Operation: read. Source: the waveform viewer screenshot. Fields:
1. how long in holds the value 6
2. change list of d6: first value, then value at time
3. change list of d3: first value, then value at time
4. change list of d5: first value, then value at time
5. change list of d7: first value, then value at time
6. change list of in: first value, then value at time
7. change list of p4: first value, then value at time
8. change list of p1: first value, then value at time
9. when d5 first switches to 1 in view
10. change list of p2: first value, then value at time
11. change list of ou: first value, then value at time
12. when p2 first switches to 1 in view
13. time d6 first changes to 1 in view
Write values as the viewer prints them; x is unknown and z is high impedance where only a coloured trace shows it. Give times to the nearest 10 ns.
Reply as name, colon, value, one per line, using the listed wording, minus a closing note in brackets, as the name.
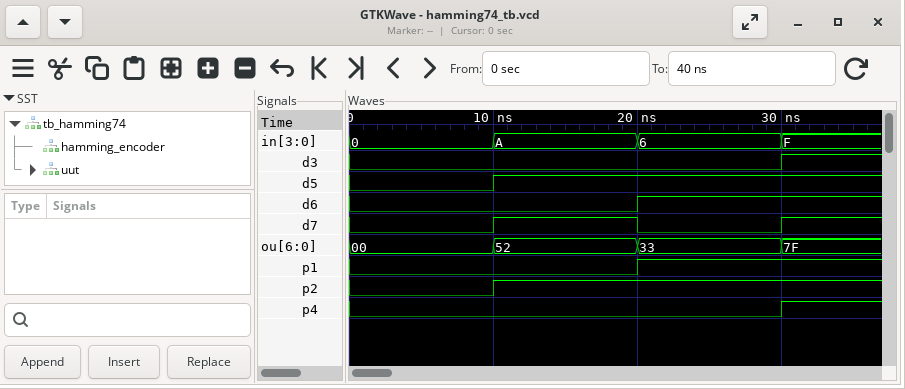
how long in holds the value 6: 10 ns
change list of d6: first value, then value at time: 0, 1 at 20 ns
change list of d3: first value, then value at time: 0, 1 at 30 ns
change list of d5: first value, then value at time: 0, 1 at 10 ns
change list of d7: first value, then value at time: 0, 1 at 10 ns, 0 at 20 ns, 1 at 30 ns
change list of in: first value, then value at time: 0, A at 10 ns, 6 at 20 ns, F at 30 ns
change list of p4: first value, then value at time: 0, 1 at 30 ns
change list of p1: first value, then value at time: 0, 1 at 20 ns
when d5 first switches to 1 in view: 10 ns
change list of p2: first value, then value at time: 0, 1 at 10 ns
change list of ou: first value, then value at time: 00, 52 at 10 ns, 33 at 20 ns, 7F at 30 ns
when p2 first switches to 1 in view: 10 ns
time d6 first changes to 1 in view: 20 ns
